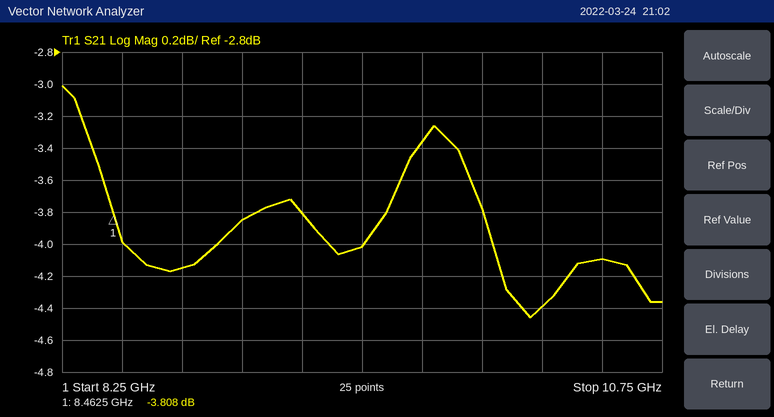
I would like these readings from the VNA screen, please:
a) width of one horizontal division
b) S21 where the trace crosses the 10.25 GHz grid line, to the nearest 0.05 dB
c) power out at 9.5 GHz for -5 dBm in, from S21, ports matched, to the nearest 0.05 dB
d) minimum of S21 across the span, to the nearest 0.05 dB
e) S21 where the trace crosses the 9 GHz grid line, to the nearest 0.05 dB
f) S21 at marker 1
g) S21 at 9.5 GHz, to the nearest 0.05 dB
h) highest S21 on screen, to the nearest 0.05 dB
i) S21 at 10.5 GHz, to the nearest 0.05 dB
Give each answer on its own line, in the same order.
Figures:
250 MHz
-4.40 dB
-9.00 dBm
-4.45 dB
-3.85 dB
-3.808 dB
-4.00 dB
-3.00 dB
-4.10 dB
